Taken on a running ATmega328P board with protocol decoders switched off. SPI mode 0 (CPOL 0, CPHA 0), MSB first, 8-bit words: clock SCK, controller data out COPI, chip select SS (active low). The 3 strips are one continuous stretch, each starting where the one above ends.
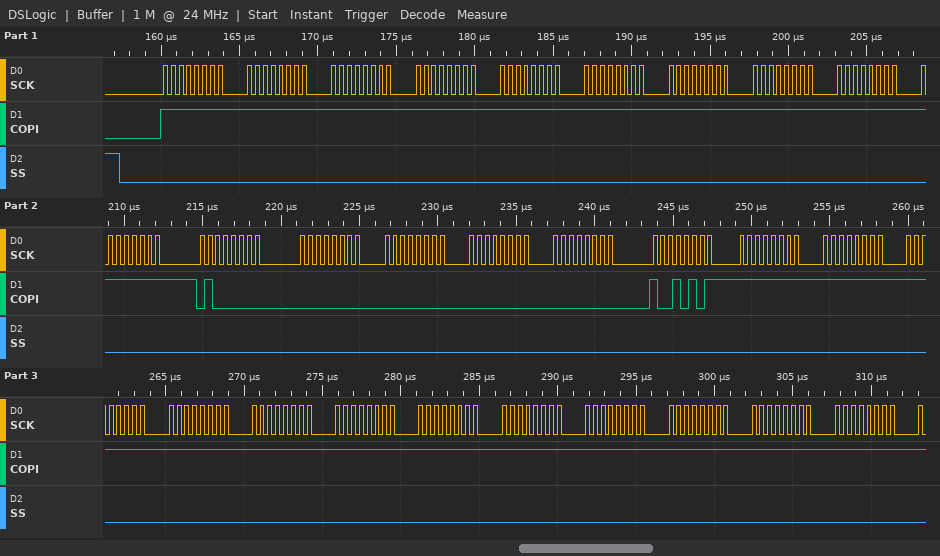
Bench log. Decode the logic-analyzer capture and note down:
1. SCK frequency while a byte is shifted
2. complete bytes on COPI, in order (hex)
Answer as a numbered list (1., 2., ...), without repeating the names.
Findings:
1. 2 MHz
2. FF FF FF FF FF FF FF FF FF FF 40 00 00 00 00 95 FF FF FF FF FF FF FF FF FF FF FF FF
